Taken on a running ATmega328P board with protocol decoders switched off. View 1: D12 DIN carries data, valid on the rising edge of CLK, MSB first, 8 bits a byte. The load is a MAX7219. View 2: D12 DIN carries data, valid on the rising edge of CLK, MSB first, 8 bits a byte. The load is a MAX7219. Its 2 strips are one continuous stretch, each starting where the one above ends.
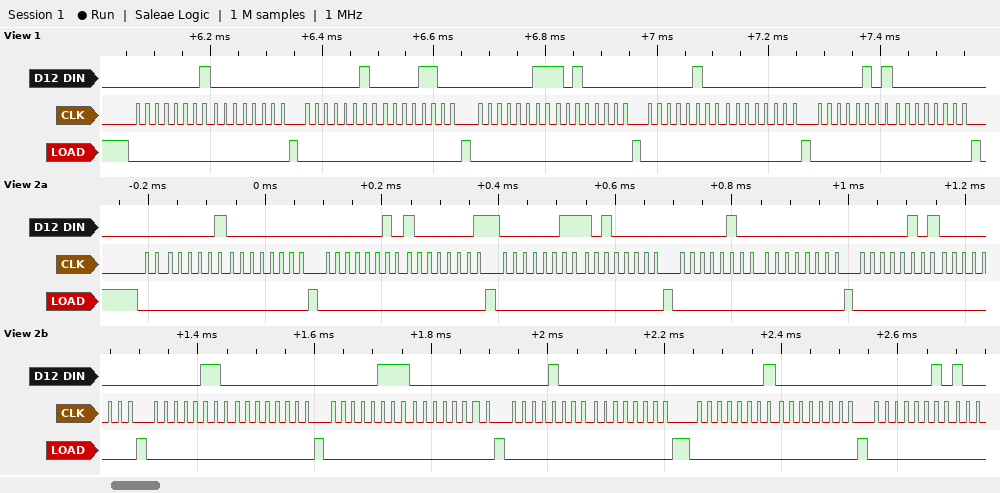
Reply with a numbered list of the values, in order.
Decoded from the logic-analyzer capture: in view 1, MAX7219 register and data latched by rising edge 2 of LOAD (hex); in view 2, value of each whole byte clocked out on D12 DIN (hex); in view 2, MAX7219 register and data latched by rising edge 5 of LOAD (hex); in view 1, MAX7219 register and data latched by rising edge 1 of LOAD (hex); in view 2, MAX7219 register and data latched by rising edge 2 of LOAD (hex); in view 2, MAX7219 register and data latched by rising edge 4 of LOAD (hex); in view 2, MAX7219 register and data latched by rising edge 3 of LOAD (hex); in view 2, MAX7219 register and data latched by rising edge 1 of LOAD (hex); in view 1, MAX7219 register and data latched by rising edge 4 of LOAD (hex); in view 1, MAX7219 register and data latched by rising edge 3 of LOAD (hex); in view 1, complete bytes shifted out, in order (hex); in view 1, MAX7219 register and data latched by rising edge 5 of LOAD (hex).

1. register 0x2, data 0x0C
2. 01 00 02 81 03 A0 04 00 05 00 06 00 07 00 08 00 01 00 02
3. register 0x5, data 0x00
4. register 0x1, data 0x00
5. register 0x2, data 0x81
6. register 0x4, data 0x00
7. register 0x3, data 0xA0
8. register 0x1, data 0x00
9. register 0x4, data 0x00
10. register 0x3, data 0xA0
11. 0x01 0x00 0x02 0x0C 0x03 0xA0 0x04 0x00 0x05 0x00
12. register 0x5, data 0x00
